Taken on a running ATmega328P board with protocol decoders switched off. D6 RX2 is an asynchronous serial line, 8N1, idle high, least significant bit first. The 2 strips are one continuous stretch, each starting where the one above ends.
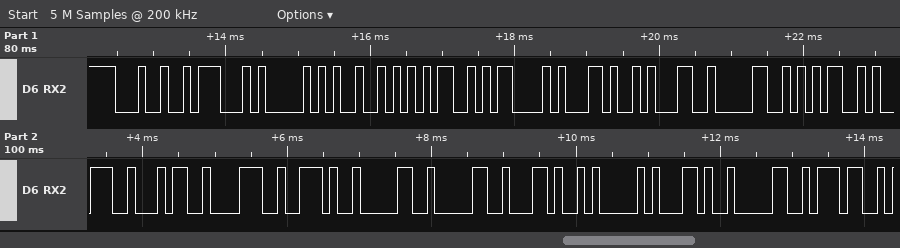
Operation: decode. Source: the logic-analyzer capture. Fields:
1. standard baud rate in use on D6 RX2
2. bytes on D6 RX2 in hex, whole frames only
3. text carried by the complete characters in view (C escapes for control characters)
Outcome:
9600 baud
24 47 50 52 4D 43 2C 31 30 35 39 34 38 2E 30 30 2C 41 2C 30 37
"$GPRMC,105948.00,A,07"
